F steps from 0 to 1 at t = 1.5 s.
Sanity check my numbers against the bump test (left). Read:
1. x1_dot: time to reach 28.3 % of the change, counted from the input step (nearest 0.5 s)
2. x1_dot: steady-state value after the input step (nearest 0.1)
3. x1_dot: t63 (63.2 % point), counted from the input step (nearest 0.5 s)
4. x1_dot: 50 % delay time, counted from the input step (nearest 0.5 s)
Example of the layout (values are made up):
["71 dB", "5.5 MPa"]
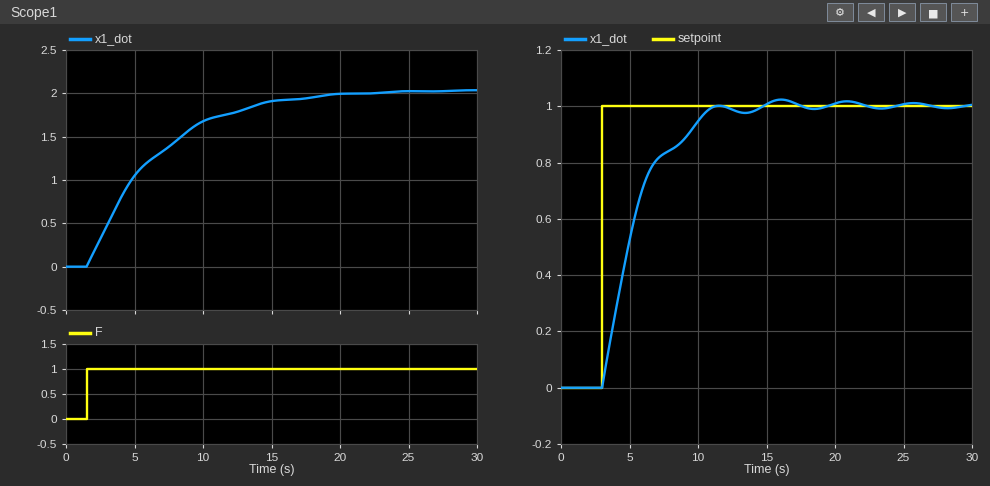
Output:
["2.0 s", "2.0", "5.0 s", "3.5 s"]
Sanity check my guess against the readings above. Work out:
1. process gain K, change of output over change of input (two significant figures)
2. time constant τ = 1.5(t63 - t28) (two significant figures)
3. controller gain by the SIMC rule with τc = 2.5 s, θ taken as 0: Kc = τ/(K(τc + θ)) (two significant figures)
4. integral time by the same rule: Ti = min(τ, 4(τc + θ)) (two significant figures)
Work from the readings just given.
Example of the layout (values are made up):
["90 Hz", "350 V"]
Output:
["2.0", "4.5 s", "0.90", "4.5 s"]
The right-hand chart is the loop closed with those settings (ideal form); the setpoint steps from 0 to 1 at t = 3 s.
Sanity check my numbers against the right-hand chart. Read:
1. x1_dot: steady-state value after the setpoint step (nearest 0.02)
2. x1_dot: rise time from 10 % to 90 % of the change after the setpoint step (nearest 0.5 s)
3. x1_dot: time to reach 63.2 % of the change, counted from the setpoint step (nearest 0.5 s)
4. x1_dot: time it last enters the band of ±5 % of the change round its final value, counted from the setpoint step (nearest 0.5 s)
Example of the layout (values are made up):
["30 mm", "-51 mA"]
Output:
["1.00", "6.0 s", "2.5 s", "7.0 s"]
